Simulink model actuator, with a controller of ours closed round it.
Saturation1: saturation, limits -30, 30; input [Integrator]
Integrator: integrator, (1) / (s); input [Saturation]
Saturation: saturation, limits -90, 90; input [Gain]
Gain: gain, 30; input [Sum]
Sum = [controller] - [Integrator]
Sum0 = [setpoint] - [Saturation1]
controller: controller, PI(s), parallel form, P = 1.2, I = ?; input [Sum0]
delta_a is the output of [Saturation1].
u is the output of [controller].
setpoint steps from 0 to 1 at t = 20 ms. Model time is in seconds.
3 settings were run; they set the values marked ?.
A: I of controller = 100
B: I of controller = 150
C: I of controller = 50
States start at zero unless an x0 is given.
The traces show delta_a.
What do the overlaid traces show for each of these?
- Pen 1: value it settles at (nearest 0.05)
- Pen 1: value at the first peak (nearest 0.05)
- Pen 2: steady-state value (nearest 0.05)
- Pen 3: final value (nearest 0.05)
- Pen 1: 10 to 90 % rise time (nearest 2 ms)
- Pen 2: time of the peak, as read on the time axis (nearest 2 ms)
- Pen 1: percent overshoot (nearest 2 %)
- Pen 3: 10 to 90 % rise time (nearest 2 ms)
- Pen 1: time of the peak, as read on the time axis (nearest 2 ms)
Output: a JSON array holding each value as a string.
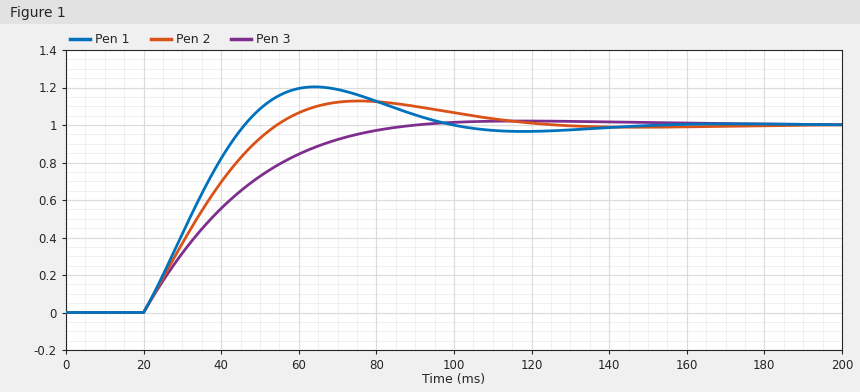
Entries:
["1.00", "1.20", "1.00", "1.00", "20 ms", "76 ms", "20 %", "44 ms", "64 ms"]
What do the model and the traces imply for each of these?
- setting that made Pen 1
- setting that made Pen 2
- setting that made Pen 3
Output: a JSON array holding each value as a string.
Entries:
["B", "A", "C"]
